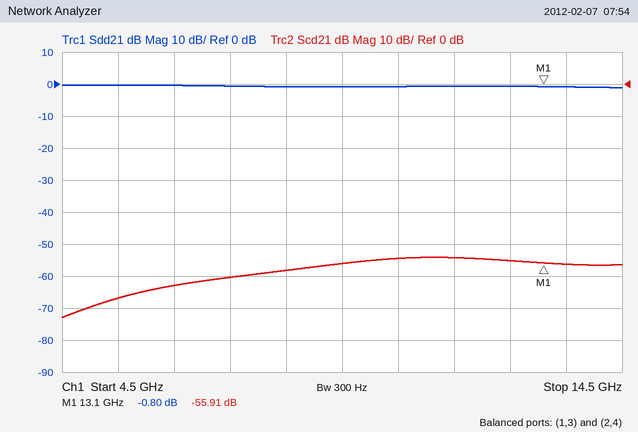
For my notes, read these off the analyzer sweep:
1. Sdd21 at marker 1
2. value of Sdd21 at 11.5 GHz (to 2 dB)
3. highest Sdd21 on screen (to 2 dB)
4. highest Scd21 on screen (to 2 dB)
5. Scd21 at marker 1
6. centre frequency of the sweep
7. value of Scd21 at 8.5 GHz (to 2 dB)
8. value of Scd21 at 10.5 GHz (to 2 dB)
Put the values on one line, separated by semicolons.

-0.80 dB; 0 dB; 0 dB; -54 dB; -55.91 dB; 9.5 GHz; -58 dB; -54 dB
